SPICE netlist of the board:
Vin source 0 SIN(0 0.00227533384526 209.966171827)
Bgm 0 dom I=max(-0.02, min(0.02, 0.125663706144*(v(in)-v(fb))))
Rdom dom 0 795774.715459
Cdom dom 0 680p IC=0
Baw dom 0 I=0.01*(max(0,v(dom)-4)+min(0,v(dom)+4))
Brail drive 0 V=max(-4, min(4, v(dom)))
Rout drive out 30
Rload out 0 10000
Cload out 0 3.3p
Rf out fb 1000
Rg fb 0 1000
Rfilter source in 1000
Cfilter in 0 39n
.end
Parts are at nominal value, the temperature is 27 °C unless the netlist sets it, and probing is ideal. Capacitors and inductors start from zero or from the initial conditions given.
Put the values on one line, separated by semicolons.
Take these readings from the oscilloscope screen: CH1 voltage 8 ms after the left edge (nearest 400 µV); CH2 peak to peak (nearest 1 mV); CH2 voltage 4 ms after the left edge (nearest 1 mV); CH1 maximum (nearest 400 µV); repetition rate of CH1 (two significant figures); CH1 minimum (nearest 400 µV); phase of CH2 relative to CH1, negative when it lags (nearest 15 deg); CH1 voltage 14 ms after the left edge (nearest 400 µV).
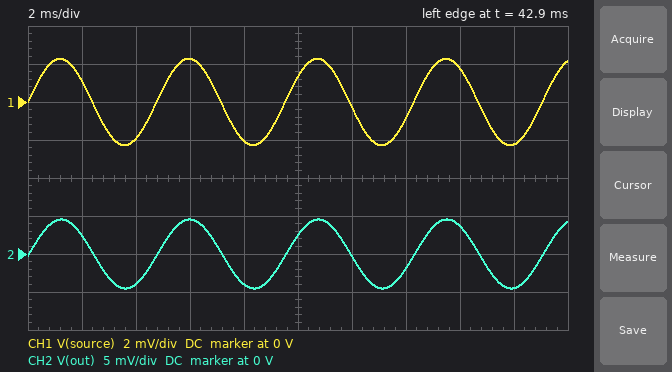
-2.0 mV; 9 mV; -4 mV; 2.4 mV; 210 Hz; -2.4 mV; 0 deg; -800 µV
